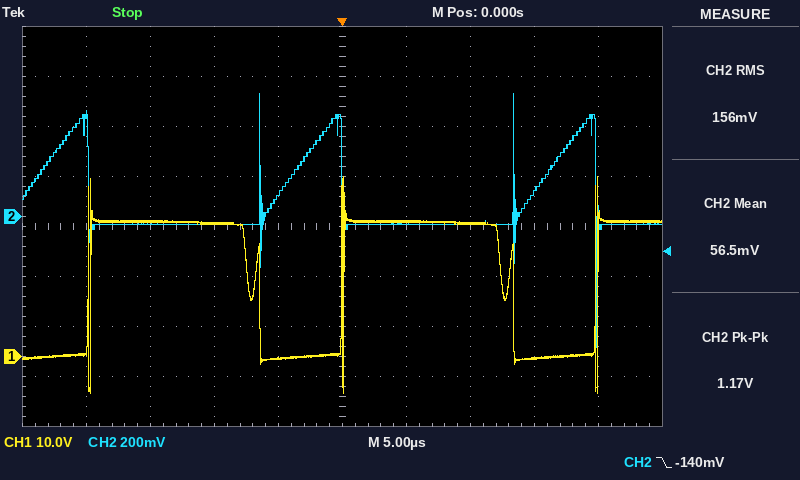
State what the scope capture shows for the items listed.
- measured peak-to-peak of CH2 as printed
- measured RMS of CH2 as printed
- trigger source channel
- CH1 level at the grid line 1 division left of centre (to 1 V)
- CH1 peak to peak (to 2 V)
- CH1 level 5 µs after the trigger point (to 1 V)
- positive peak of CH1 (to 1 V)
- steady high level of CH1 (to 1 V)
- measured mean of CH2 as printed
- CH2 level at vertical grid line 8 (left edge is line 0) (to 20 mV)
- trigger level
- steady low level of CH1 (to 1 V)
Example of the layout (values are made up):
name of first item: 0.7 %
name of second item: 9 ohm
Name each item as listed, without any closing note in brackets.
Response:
measured peak-to-peak of CH2 as printed: 1.17 V
measured RMS of CH2 as printed: 156 mV
trigger source channel: CH2
CH1 level at the grid line 1 division left of centre: 0 V
CH1 peak to peak: 44 V
CH1 level 5 µs after the trigger point: 27 V
positive peak of CH1: 36 V
steady high level of CH1: 27 V
measured mean of CH2 as printed: 56.5 mV
CH2 level at vertical grid line 8 (left edge is line 0): 100 mV
trigger level: -140 mV
steady low level of CH1: 0 V
